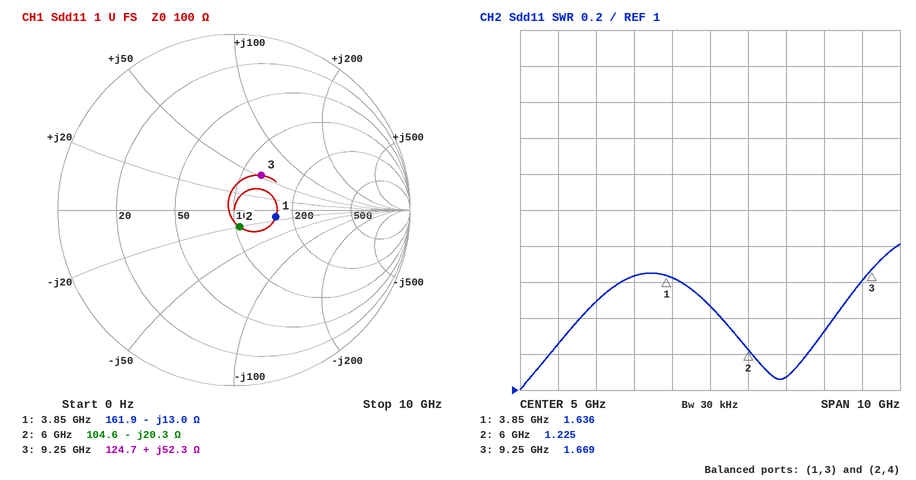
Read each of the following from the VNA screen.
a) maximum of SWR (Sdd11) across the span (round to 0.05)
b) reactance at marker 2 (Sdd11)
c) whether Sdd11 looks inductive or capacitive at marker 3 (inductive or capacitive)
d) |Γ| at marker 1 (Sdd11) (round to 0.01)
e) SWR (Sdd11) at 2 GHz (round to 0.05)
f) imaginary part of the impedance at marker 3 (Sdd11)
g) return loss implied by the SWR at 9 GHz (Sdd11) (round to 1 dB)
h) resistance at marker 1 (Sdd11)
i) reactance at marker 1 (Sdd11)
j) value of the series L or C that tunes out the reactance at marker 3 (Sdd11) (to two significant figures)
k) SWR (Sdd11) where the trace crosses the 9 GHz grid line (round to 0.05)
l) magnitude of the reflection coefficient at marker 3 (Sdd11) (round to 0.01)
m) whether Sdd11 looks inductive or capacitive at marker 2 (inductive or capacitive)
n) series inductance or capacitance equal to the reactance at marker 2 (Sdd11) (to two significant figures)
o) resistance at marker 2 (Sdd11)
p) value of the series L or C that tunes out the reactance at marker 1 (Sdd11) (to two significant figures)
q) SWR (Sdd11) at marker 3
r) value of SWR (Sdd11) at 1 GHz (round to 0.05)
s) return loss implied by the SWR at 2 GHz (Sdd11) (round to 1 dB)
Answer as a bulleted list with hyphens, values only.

- 1.80
- -20.3 Ω
- inductive
- 0.24
- 1.50
- +52.3 Ω
- 13 dB
- 161.9 Ω
- -13.0 Ω
- 330 fF
- 1.60
- 0.25
- capacitive
- 1.3 pF
- 104.6 Ω
- 540 pH
- 1.669
- 1.25
- 14 dB
